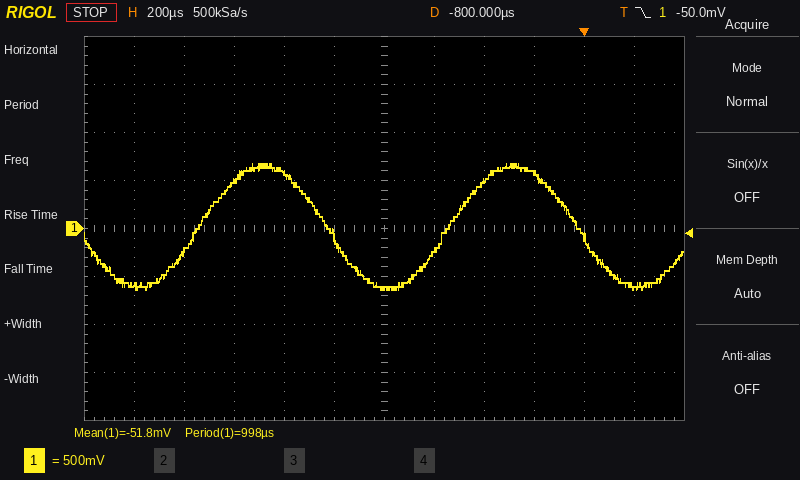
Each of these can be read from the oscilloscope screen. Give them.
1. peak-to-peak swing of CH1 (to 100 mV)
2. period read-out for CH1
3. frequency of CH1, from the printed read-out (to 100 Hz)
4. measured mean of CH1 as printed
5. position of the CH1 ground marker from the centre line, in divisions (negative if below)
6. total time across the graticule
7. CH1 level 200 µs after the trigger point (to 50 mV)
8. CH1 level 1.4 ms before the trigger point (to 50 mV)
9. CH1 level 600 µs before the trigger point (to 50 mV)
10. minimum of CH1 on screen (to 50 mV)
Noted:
1.30 V
998 µs
1.0 kHz
-51.8 mV
0.0 div
2.4 ms
-600 mV
500 mV
-250 mV
-650 mV
